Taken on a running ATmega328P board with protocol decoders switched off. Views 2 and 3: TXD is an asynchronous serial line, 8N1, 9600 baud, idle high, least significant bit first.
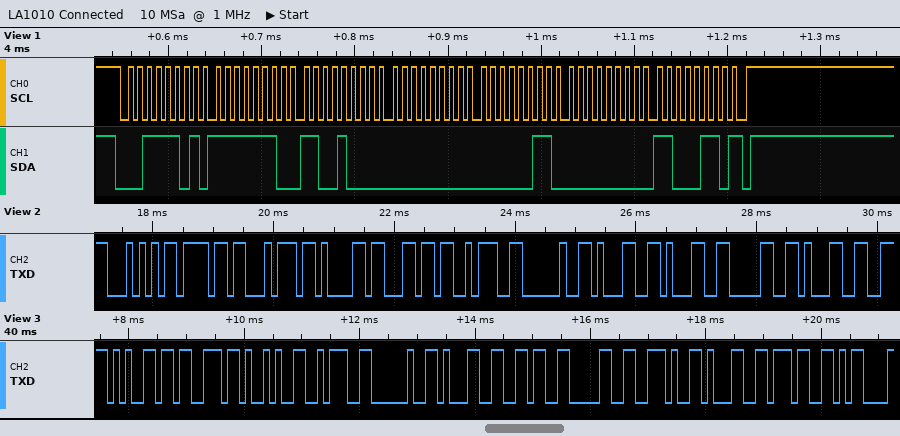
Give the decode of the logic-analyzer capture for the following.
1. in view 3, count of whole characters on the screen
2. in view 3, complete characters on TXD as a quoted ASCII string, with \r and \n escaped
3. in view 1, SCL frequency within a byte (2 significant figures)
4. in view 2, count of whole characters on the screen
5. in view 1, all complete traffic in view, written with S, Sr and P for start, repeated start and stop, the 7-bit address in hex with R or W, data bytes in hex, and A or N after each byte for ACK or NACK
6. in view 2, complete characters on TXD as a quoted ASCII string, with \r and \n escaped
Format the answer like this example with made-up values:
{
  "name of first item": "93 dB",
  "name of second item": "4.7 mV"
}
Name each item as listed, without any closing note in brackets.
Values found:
{
  "in view 3, count of whole characters on the screen": "12",
  "in view 3, complete characters on TXD as a quoted ASCII string, with \\r and \\n escaped": "\"es): 160.17\\r\"",
  "in view 1, SCL frequency within a byte": "100 kHz",
  "in view 2, count of whole characters on the screen": "11",
  "in view 1, all complete traffic in view, written with S, Sr and P for start, repeated start and stop, the 7-bit address in hex with R or W, data bytes in hex, and A or N after each byte for ACK or NACK": "S 1ER A FE A C8 A 00 A 03 A 00 A C6 N P",
  "in view 2, complete characters on TXD as a quoted ASCII string, with \\r and \\n escaped": "\"Total: 1101\""
}
